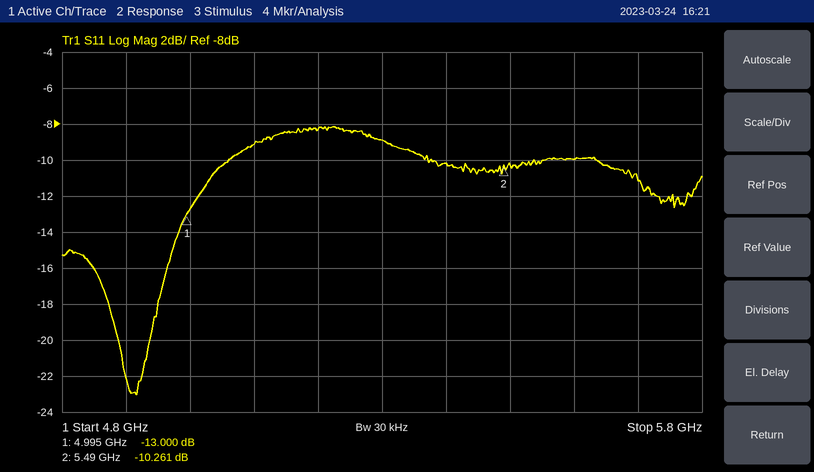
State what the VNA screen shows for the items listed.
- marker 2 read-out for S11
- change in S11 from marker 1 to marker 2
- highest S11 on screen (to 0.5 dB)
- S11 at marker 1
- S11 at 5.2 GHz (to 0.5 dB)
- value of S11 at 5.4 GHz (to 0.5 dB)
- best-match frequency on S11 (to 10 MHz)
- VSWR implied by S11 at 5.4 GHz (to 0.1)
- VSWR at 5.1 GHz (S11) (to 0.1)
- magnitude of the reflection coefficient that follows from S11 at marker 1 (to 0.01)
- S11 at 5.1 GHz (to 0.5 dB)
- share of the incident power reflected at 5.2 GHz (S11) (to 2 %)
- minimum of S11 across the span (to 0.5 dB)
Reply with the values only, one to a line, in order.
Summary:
-10.261 dB
2.739 dB
-8.0 dB
-13.000 dB
-8.5 dB
-10.0 dB
4.92 GHz
1.9
2.1
0.22
-9.0 dB
14 %
-23.0 dB
